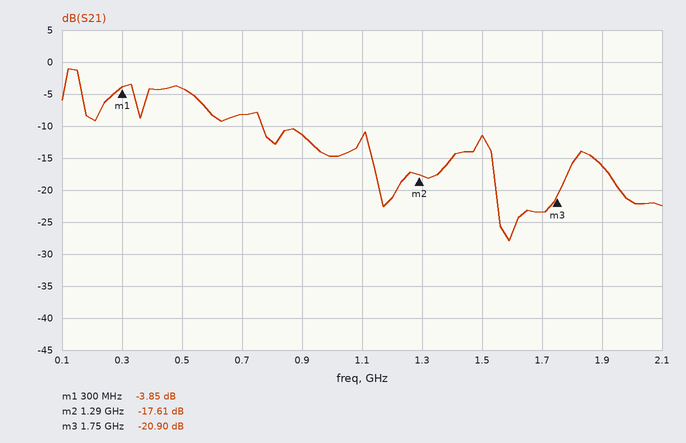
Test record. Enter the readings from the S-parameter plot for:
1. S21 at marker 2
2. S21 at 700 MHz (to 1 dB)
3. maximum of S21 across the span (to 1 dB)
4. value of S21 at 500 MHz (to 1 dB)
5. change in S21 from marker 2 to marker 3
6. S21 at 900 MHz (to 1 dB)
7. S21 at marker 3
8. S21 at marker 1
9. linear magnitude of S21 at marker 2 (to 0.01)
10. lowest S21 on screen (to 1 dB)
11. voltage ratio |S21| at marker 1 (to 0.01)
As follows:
-17.61 dB
-8 dB
-1 dB
-4 dB
-3.29 dB
-11 dB
-20.90 dB
-3.85 dB
0.13
-28 dB
0.64
